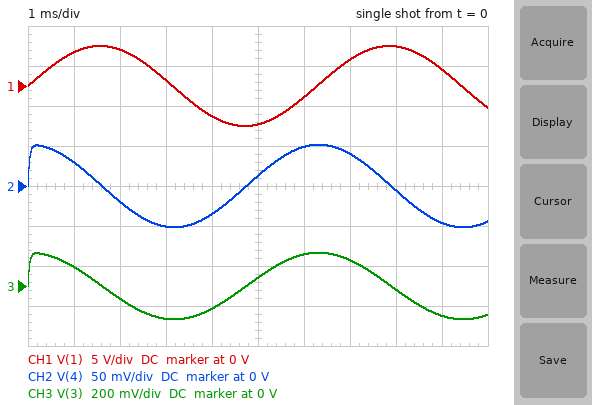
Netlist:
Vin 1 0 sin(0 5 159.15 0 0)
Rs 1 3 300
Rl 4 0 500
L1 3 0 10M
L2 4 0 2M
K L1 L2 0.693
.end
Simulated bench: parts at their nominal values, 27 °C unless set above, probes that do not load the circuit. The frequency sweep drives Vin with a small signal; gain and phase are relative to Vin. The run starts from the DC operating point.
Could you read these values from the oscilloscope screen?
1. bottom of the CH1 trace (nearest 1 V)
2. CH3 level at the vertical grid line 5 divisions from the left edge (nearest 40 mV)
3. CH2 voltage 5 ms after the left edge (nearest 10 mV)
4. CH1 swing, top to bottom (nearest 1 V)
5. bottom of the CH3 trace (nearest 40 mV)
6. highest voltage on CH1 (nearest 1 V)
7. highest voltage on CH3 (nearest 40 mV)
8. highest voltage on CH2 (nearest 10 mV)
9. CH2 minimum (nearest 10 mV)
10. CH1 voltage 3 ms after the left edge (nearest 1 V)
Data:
-5 V
40 mV
10 mV
10 V
-160 mV
5 V
160 mV
50 mV
-50 mV
1 V
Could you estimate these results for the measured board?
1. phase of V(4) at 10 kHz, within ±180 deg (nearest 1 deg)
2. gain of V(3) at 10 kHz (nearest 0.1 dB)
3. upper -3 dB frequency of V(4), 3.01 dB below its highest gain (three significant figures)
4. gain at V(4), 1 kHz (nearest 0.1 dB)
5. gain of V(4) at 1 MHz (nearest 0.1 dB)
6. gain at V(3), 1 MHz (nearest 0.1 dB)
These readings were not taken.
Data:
17 deg
-1.3 dB
89.8 kHz
-24.0 dB
-32.5 dB
0 dB
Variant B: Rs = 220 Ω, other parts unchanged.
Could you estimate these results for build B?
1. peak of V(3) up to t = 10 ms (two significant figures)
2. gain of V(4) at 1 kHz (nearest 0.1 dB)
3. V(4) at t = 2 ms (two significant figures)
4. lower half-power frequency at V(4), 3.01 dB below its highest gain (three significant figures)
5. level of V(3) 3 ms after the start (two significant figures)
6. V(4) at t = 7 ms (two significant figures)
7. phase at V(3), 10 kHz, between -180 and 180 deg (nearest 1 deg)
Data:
230 mV
-21.4 dB
-26 mV
3.10 kHz
-220 mV
55 mV
19 deg
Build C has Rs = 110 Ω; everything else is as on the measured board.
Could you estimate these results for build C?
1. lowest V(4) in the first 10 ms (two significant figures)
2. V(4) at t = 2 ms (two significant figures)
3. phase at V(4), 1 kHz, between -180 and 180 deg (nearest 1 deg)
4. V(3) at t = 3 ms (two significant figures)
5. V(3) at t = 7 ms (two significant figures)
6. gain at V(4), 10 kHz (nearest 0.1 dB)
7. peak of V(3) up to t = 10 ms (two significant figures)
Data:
-140 mV
-46 mV
59 deg
-440 mV
370 mV
-10.6 dB
450 mV
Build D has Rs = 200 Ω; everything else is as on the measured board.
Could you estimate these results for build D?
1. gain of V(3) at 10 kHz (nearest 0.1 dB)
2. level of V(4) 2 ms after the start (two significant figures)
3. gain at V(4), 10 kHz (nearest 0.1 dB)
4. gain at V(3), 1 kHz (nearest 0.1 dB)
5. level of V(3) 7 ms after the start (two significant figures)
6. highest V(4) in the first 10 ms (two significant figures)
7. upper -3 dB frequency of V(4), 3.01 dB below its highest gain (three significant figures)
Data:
-0.7 dB
-28 mV
-11.0 dB
-10.5 dB
200 mV
77 mV
85.5 kHz
